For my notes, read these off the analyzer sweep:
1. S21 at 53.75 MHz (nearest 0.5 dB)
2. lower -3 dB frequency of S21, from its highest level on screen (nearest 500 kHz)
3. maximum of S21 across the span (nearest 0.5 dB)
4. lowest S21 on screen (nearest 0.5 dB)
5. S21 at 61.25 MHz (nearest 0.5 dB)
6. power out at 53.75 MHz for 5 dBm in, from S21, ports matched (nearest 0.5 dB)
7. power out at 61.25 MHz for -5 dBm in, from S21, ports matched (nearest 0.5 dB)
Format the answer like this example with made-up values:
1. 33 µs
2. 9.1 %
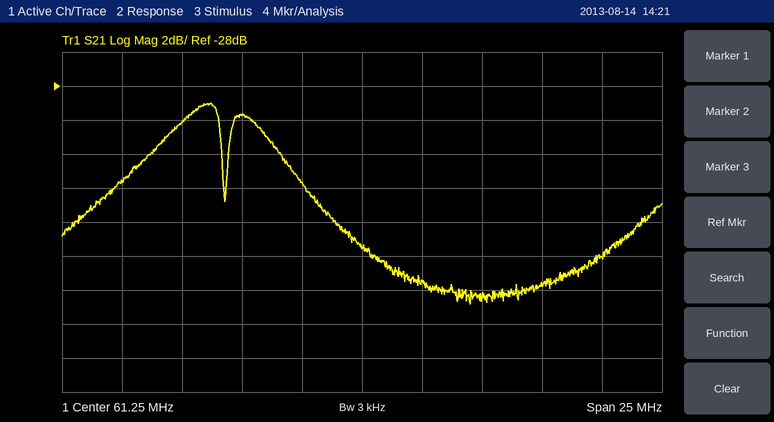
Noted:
1. -30.0 dB
2. 52.5 MHz
3. -29.0 dB
4. -41.0 dB
5. -37.5 dB
6. -25.0 dBm
7. -42.5 dBm
